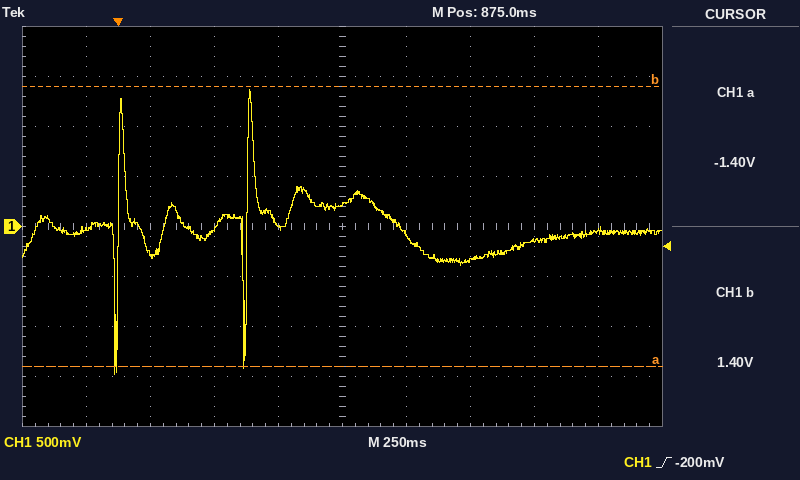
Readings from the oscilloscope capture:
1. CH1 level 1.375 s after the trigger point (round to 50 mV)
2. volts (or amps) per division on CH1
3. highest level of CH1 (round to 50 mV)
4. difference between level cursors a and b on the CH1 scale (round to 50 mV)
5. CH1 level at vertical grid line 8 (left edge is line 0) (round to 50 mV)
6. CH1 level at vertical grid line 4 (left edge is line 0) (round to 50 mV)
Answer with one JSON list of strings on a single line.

["-350 mV", "500 mV", "1.35 V", "2.80 V", "-150 mV", "0 mV"]
